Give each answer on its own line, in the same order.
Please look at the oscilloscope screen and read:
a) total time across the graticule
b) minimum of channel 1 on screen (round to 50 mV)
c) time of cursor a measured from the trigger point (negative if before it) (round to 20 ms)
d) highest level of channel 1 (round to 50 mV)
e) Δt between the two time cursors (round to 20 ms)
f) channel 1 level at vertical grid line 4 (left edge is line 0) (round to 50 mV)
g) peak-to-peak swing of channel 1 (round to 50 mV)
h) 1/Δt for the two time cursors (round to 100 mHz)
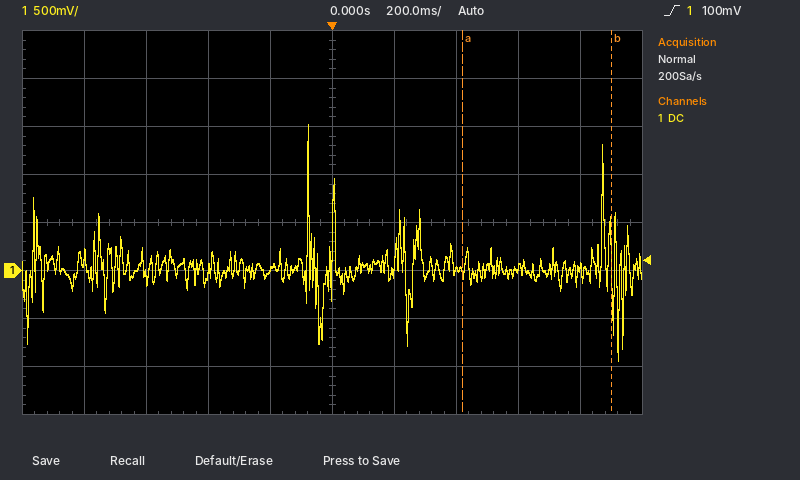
2 s
-950 mV
+420 ms
1.50 V
480 ms
0 mV
2.45 V
2.1 Hz
